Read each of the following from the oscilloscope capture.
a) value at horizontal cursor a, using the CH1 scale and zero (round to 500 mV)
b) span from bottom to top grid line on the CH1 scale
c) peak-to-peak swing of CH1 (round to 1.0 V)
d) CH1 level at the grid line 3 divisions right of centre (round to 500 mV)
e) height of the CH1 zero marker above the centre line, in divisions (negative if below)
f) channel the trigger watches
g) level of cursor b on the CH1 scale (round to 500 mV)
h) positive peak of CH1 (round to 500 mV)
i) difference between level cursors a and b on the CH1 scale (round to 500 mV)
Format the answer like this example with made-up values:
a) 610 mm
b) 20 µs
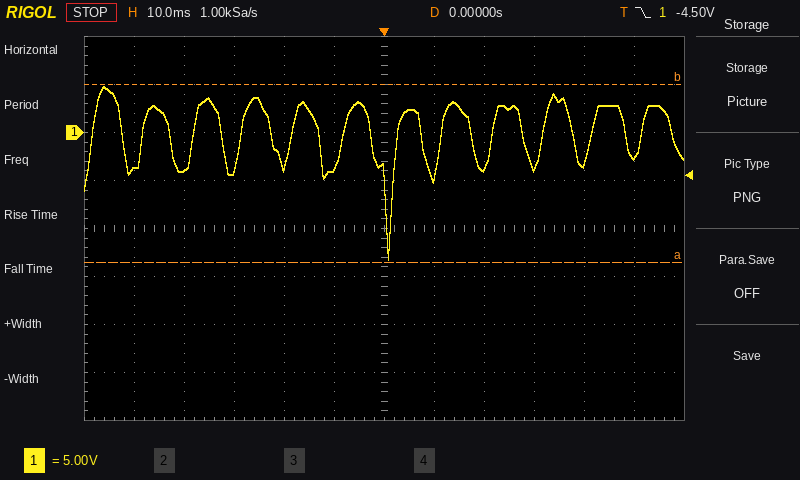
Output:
a) -13.5 V
b) 40 V
c) 18.0 V
d) -3.5 V
e) +2.0 div
f) CH1
g) 5.0 V
h) 5.0 V
i) 18.5 V
